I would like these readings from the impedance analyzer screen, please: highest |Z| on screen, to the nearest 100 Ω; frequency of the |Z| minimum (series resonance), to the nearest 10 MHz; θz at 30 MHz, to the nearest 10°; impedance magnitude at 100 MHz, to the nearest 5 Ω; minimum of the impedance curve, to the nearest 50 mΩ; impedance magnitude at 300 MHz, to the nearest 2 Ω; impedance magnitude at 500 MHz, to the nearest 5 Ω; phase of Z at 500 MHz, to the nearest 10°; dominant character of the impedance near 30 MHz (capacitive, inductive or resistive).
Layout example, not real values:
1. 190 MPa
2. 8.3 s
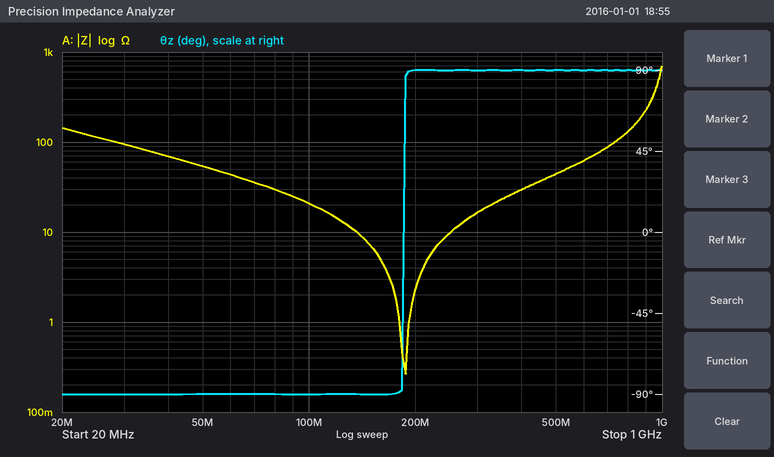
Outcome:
1. 700 Ω
2. 190 MHz
3. -90°
4. 20 Ω
5. 250 mΩ
6. 16 Ω
7. 45 Ω
8. 90°
9. capacitive
